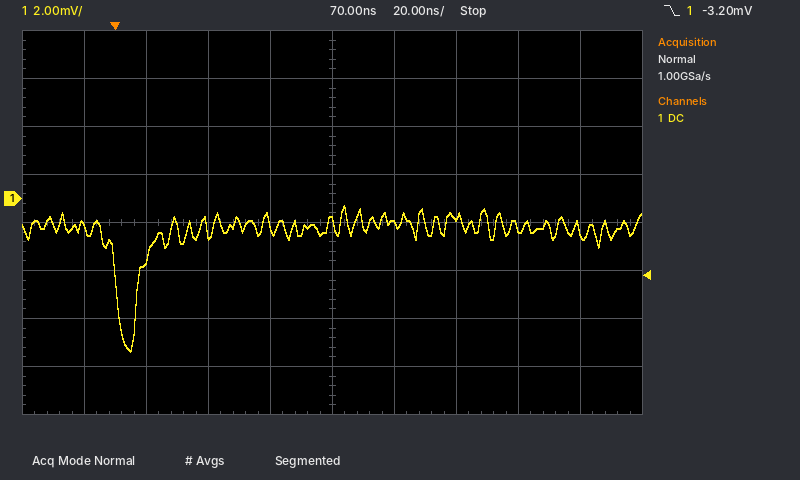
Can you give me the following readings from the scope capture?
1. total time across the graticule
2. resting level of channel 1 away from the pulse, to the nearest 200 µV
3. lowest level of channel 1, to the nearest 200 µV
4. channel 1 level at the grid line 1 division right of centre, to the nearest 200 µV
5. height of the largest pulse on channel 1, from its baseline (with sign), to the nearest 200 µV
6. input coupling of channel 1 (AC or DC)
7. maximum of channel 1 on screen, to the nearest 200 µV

200 ns
-1.2 mV
-6.4 mV
-1.0 mV
-5.2 mV
DC
-200 µV
